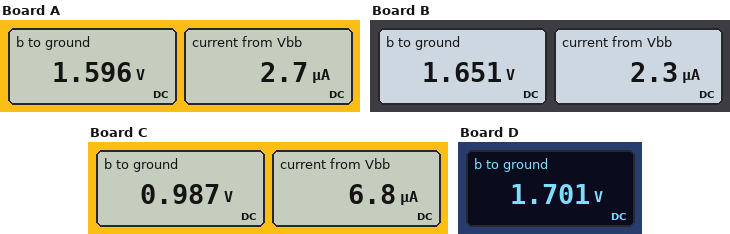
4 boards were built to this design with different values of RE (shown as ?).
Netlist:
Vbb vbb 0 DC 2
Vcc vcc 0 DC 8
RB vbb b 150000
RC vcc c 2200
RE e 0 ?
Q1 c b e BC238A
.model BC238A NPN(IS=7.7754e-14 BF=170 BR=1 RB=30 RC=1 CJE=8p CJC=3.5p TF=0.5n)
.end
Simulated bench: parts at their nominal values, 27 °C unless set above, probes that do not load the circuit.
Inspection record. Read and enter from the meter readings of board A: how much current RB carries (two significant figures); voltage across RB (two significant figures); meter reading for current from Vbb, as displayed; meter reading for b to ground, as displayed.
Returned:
2.7 µA
400 mV
2.7 µA
1.596 V
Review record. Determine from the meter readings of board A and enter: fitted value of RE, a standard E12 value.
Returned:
2.2 kΩ
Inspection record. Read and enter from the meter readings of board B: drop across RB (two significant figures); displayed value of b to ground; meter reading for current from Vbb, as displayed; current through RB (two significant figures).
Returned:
350 mV
1.651 V
2.3 µA
2.3 µA
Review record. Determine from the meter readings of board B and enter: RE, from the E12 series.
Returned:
2.7 kΩ
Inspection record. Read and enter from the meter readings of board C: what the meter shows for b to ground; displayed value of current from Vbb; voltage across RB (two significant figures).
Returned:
0.987 V
6.8 µA
1.0 V
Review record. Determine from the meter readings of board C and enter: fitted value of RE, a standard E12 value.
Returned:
330 Ω
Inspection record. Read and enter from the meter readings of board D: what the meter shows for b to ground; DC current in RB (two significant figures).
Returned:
1.701 V
2.0 µA
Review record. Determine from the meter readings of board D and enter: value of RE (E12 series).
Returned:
3.3 kΩ
